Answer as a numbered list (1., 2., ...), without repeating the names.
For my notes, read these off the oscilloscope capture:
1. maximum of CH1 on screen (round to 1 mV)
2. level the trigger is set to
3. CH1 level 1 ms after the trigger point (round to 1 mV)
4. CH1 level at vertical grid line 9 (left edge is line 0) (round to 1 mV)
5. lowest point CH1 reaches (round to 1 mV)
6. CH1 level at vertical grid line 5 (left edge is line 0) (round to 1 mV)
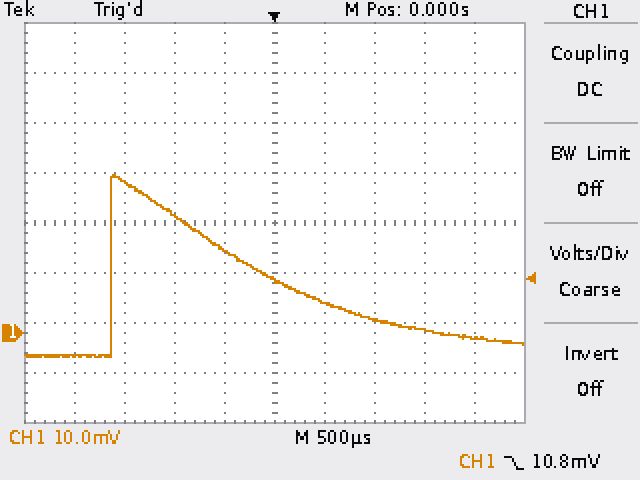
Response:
1. 32 mV
2. 10.8 mV
3. 3 mV
4. -1 mV
5. -5 mV
6. 11 mV
